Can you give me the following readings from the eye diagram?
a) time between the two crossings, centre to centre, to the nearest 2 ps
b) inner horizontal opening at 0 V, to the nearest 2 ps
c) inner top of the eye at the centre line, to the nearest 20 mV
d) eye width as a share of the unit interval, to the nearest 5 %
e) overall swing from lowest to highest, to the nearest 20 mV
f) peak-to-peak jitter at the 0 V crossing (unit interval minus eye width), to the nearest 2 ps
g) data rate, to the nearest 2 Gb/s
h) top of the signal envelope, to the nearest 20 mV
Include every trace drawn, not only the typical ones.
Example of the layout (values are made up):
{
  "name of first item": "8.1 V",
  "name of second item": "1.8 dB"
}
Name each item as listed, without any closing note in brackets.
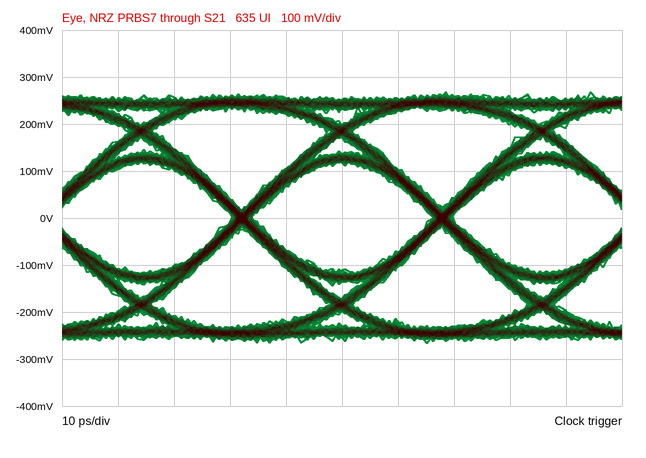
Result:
{
  "time between the two crossings, centre to centre, to the nearest 2 ps": "36 ps",
  "inner horizontal opening at 0 V, to the nearest 2 ps": "32 ps",
  "inner top of the eye at the centre line, to the nearest 20 mV": "120 mV",
  "eye width as a share of the unit interval, to the nearest 5 %": "90 %",
  "overall swing from lowest to highest, to the nearest 20 mV": "540 mV",
  "peak-to-peak jitter at the 0 V crossing (unit interval minus eye width), to the nearest 2 ps": "4 ps",
  "data rate, to the nearest 2 Gb/s": "28 Gb/s",
  "top of the signal envelope, to the nearest 20 mV": "260 mV"
}
